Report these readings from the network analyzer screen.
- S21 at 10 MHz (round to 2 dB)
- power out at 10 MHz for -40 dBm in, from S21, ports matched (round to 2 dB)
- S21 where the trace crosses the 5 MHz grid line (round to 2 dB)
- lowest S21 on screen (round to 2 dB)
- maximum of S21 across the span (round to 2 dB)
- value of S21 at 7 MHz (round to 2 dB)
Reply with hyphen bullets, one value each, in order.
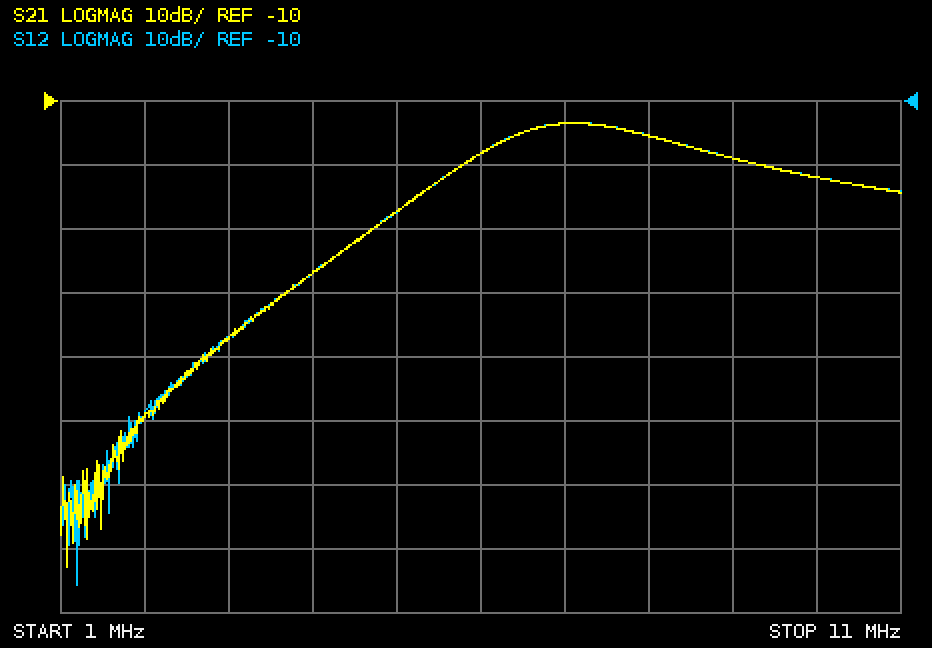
- -22 dB
- -62 dBm
- -28 dB
- -82 dB
- -14 dB
- -14 dB
